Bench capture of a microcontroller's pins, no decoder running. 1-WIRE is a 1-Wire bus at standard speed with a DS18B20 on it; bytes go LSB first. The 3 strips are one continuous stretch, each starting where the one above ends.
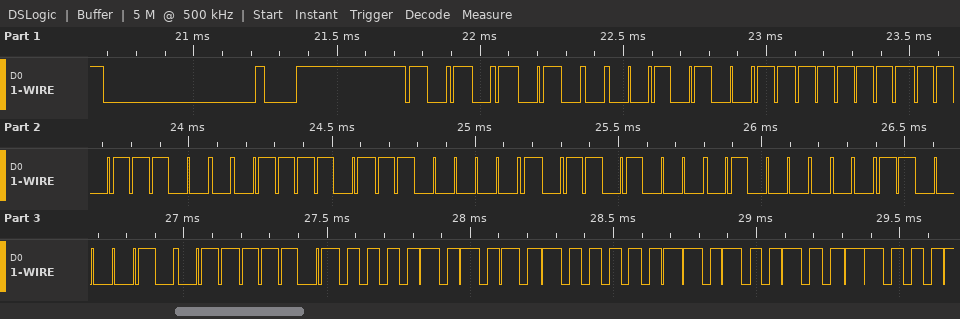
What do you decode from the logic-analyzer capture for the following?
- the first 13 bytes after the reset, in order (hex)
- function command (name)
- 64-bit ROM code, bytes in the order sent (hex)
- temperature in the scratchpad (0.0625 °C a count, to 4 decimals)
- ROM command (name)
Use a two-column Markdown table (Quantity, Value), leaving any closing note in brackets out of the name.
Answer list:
| Quantity | Value |
|---|---|
| the first 13 bytes after the reset, in order | 55 28 FF 3B BC 83 16 02 43 BE 50 05 4B |
| function command | Read Scratchpad |
| 64-bit ROM code, bytes in the order sent | 28 FF 3B BC 83 16 02 43 |
| temperature in the scratchpad | 85.0000 °C |
| ROM command | Match ROM |
